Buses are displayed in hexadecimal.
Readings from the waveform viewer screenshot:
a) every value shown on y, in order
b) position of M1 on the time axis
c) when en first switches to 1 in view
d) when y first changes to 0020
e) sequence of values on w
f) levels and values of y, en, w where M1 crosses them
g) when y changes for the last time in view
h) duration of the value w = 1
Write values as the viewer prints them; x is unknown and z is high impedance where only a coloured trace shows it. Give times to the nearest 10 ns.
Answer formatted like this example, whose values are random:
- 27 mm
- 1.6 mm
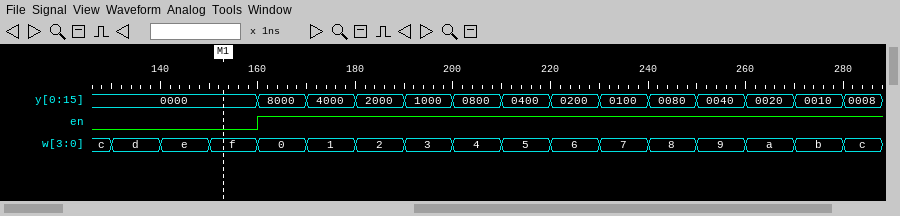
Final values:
- 0000, 8000, 4000, 2000, 1000, 0800, 0400, 0200, 0100, 0080, 0040, 0020, 0010, 0008
- 150 ns
- 160 ns
- 260 ns
- c, d, e, f, 0, 1, 2, 3, 4, 5, 6, 7, 8, 9, a, b, c
- y=0000, en=0, w=f
- 280 ns
- 10 ns
